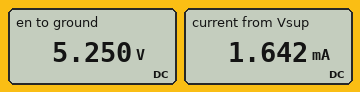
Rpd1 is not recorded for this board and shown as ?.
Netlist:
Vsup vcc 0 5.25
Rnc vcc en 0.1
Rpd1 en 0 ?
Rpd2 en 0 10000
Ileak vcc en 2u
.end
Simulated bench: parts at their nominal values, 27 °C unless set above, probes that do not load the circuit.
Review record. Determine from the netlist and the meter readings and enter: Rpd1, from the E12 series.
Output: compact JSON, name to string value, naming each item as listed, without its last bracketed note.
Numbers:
{"Rpd1, from the E12 series": "4.7 kΩ"}
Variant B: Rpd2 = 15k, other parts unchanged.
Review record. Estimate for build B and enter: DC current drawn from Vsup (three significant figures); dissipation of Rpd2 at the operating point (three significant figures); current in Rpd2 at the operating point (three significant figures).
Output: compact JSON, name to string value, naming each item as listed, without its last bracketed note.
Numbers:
{"DC current drawn from Vsup": "1.47 mA", "dissipation of Rpd2 at the operating point": "1.84 mW", "current in Rpd2 at the operating point": "350 µA"}
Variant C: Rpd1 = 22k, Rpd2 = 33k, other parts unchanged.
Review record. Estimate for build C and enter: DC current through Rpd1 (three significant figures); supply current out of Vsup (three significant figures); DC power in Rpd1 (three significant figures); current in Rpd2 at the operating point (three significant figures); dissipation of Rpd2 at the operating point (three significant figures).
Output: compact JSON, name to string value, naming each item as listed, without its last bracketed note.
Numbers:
{"DC current through Rpd1": "239 µA", "supply current out of Vsup": "398 µA", "DC power in Rpd1": "1.25 mW", "current in Rpd2 at the operating point": "159 µA", "dissipation of Rpd2 at the operating point": "835 µW"}
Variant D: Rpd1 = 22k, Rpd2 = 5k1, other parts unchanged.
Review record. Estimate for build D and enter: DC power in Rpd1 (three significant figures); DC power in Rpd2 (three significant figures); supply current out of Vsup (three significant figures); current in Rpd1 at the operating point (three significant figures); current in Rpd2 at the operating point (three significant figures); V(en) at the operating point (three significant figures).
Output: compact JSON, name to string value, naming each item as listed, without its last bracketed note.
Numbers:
{"DC power in Rpd1": "1.25 mW", "DC power in Rpd2": "5.40 mW", "supply current out of Vsup": "1.27 mA", "current in Rpd1 at the operating point": "239 µA", "current in Rpd2 at the operating point": "1.03 mA", "V(en) at the operating point": "5.25 V"}
